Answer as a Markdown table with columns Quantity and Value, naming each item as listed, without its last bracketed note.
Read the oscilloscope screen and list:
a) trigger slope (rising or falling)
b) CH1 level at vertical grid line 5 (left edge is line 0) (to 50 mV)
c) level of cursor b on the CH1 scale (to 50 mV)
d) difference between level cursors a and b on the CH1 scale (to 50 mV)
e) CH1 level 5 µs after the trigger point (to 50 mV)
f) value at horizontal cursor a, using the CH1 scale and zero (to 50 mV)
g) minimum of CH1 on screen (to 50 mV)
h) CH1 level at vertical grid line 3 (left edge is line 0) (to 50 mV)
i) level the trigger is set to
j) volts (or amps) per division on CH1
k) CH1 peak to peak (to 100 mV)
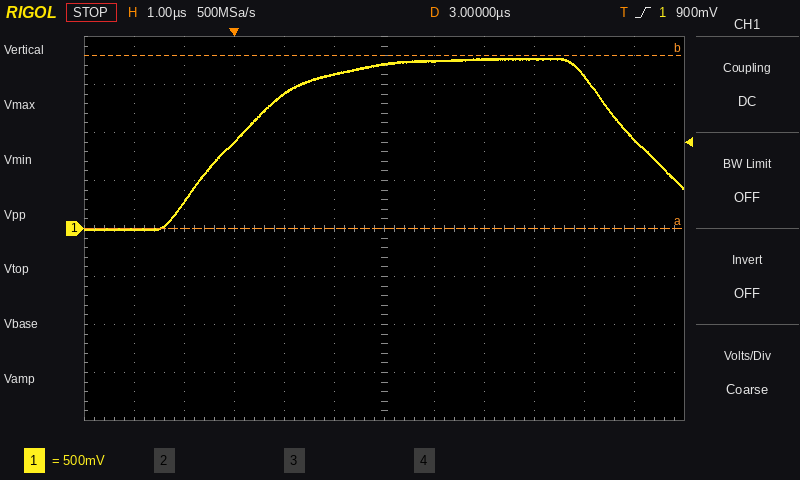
| Quantity | Value |
|---|---|
| trigger slope | rising |
| CH1 level at vertical grid line 5 (left edge is line 0) | 1.60 V |
| level of cursor b on the CH1 scale | 1.80 V |
| difference between level cursors a and b on the CH1 scale | 1.80 V |
| CH1 level 5 µs after the trigger point | 1.75 V |
| value at horizontal cursor a, using the CH1 scale and zero | 0 mV |
| minimum of CH1 on screen | 0 mV |
| CH1 level at vertical grid line 3 (left edge is line 0) | 900 mV |
| level the trigger is set to | 900 mV |
| volts (or amps) per division on CH1 | 500 mV |
| CH1 peak to peak | 1.80 V |
